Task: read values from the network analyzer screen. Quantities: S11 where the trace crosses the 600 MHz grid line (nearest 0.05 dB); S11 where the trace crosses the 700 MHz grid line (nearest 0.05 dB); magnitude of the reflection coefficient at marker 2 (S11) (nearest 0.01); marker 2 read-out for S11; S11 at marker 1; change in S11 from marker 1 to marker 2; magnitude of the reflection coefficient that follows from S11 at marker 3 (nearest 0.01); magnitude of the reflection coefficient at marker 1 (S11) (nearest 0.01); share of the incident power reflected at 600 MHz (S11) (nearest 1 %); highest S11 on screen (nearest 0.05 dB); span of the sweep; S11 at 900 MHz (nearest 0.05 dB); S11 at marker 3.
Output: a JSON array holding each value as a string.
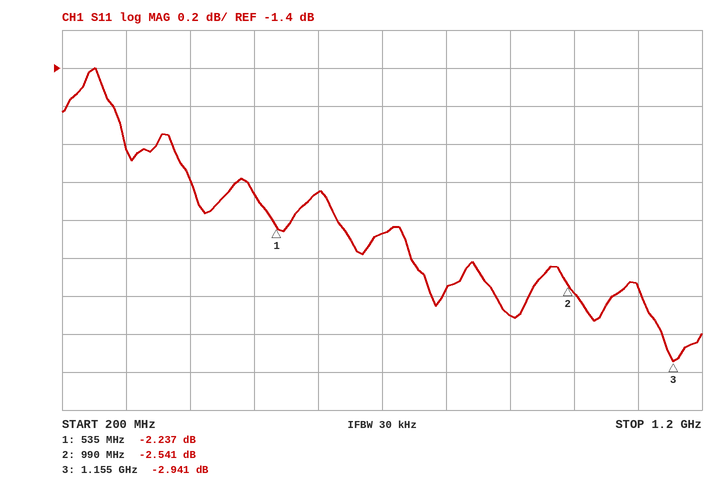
["-2.05 dB", "-2.25 dB", "0.75", "-2.541 dB", "-2.237 dB", "-0.304 dB", "0.71", "0.77", "62 %", "-1.40 dB", "1 GHz", "-2.70 dB", "-2.941 dB"]
